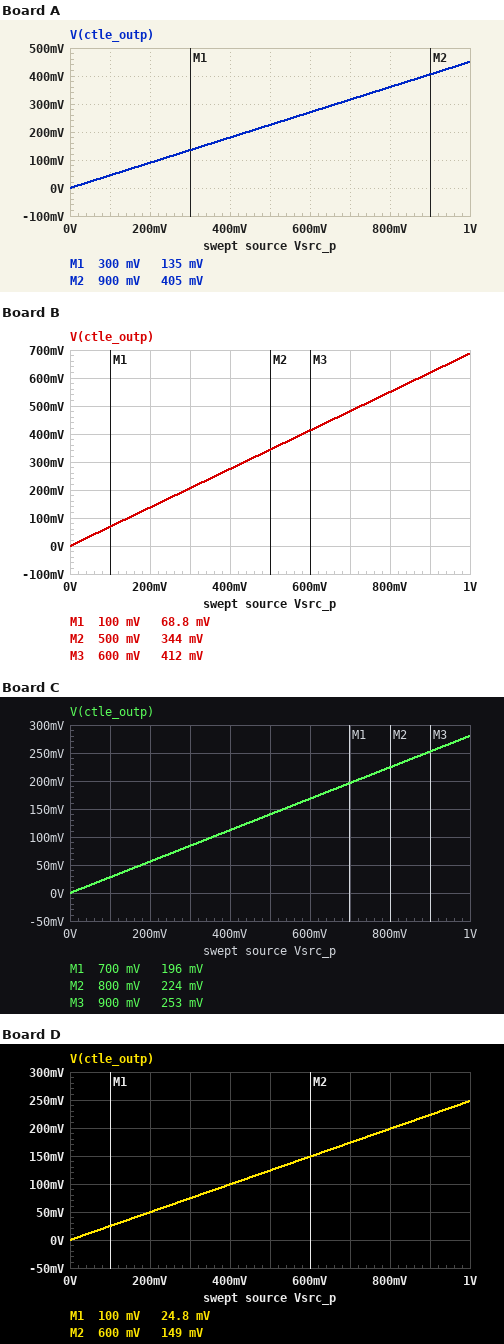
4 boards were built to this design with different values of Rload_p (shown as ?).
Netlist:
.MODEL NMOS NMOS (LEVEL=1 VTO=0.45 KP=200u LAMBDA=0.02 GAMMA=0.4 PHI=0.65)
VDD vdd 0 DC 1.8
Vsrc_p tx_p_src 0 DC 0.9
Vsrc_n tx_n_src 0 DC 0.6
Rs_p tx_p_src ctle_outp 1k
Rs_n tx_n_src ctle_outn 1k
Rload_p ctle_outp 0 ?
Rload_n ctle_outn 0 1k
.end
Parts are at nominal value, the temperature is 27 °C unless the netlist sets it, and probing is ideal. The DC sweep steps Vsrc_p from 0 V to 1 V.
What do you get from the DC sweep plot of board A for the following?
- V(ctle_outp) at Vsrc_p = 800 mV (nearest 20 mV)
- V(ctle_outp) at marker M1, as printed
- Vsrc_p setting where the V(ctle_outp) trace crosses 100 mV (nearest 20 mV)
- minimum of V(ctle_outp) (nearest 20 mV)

360 mV
135 mV
220 mV
0 V
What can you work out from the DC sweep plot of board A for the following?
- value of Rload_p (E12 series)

820 Ω
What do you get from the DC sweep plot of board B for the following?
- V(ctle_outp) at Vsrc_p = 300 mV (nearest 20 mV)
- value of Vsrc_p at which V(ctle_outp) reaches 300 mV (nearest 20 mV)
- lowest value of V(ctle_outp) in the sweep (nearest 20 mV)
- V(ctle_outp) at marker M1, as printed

200 mV
440 mV
0 V
68.8 mV
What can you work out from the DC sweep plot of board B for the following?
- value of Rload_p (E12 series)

2.2 kΩ
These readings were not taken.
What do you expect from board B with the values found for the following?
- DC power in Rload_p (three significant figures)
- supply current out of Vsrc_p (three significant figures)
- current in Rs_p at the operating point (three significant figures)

174 µW
281 µA
281 µA
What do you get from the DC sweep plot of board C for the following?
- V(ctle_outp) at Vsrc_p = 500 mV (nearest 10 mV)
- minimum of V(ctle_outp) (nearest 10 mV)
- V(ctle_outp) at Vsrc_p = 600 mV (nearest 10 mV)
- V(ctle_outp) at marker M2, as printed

140 mV
0 V
170 mV
224 mV
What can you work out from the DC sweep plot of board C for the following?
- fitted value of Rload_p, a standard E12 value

390 Ω
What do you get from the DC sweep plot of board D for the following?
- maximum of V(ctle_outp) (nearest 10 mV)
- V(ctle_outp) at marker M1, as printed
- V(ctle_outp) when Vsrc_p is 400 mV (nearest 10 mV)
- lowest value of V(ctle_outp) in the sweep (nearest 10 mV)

250 mV
24.8 mV
100 mV
0 V
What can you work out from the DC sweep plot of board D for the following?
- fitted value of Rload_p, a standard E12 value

330 Ω
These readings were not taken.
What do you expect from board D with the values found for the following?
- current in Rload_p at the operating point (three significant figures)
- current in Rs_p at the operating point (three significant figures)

677 µA
677 µA
